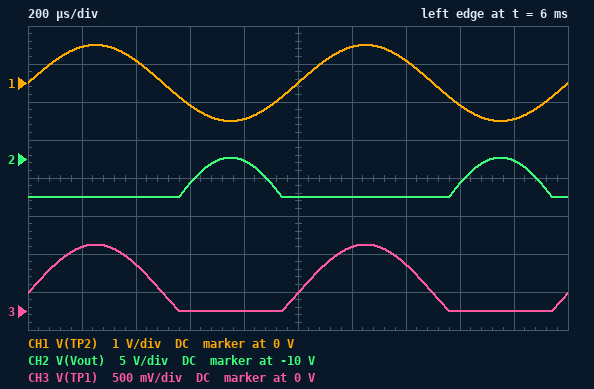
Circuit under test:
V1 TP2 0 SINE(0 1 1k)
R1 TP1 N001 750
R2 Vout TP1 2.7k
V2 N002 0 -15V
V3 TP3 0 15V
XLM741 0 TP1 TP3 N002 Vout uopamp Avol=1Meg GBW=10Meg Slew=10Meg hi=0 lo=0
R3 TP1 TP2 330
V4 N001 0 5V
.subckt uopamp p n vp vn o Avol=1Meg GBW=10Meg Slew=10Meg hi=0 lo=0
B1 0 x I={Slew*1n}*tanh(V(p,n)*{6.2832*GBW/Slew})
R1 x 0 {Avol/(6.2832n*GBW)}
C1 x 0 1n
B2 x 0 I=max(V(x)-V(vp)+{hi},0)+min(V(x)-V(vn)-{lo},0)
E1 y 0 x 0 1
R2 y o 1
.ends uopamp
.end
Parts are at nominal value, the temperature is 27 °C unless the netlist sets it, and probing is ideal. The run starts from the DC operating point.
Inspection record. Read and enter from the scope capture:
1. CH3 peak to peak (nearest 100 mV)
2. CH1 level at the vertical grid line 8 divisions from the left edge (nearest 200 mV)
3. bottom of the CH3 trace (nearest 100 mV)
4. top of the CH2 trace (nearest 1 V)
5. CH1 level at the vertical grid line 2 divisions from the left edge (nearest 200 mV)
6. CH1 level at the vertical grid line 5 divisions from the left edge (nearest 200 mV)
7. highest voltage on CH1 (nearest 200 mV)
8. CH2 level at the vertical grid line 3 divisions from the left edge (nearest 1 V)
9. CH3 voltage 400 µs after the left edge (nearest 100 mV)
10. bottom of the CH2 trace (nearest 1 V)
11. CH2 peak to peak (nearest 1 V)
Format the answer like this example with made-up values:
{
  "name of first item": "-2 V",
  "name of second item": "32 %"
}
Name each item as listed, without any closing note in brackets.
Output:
{
  "CH3 peak to peak": "900 mV",
  "CH1 level at the vertical grid line 8 divisions from the left edge": "-600 mV",
  "bottom of the CH3 trace": "0 V",
  "top of the CH2 trace": "-10 V",
  "CH1 level at the vertical grid line 2 divisions from the left edge": "600 mV",
  "CH1 level at the vertical grid line 5 divisions from the left edge": "0 V",
  "highest voltage on CH1": "1.0 V",
  "CH2 level at the vertical grid line 3 divisions from the left edge": "-13 V",
  "CH3 voltage 400 µs after the left edge": "600 mV",
  "bottom of the CH2 trace": "-15 V",
  "CH2 peak to peak": "5 V"
}
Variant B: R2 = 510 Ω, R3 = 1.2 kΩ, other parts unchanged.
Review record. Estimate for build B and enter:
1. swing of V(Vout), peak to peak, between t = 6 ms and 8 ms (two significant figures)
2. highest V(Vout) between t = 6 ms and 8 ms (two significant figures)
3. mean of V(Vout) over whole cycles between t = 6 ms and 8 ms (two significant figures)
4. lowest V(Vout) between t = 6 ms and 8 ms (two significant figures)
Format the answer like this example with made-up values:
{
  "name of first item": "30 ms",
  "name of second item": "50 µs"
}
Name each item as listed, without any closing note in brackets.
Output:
{
  "swing of V(Vout), peak to peak, between t = 6 ms and 8 ms": "850 mV",
  "highest V(Vout) between t = 6 ms and 8 ms": "-3.0 V",
  "mean of V(Vout) over whole cycles between t = 6 ms and 8 ms": "-3.4 V",
  "lowest V(Vout) between t = 6 ms and 8 ms": "-3.8 V"
}
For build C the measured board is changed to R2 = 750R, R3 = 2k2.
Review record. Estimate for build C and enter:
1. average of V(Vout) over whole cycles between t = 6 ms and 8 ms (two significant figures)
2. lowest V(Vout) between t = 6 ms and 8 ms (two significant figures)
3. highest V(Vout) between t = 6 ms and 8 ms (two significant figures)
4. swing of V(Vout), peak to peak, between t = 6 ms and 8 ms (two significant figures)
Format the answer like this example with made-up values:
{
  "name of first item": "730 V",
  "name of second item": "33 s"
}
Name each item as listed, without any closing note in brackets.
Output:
{
  "average of V(Vout) over whole cycles between t = 6 ms and 8 ms": "-5.0 V",
  "lowest V(Vout) between t = 6 ms and 8 ms": "-5.3 V",
  "highest V(Vout) between t = 6 ms and 8 ms": "-4.7 V",
  "swing of V(Vout), peak to peak, between t = 6 ms and 8 ms": "680 mV"
}
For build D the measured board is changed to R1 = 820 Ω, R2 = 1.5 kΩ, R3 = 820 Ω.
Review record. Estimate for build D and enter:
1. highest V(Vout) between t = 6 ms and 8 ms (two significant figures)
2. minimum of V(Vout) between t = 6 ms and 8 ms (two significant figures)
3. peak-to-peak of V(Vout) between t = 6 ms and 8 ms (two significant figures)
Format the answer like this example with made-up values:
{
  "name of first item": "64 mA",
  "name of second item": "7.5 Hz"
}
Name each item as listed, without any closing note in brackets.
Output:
{
  "highest V(Vout) between t = 6 ms and 8 ms": "-7.3 V",
  "minimum of V(Vout) between t = 6 ms and 8 ms": "-11 V",
  "peak-to-peak of V(Vout) between t = 6 ms and 8 ms": "3.7 V"
}
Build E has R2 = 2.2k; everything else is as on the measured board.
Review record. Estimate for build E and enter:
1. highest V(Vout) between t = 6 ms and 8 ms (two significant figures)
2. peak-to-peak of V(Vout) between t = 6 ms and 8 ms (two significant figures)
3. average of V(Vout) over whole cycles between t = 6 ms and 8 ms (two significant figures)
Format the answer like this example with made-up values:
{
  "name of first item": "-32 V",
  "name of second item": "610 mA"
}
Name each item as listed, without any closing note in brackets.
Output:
{
  "highest V(Vout) between t = 6 ms and 8 ms": "-8.0 V",
  "peak-to-peak of V(Vout) between t = 6 ms and 8 ms": "7.0 V",
  "average of V(Vout) over whole cycles between t = 6 ms and 8 ms": "-13 V"
}
